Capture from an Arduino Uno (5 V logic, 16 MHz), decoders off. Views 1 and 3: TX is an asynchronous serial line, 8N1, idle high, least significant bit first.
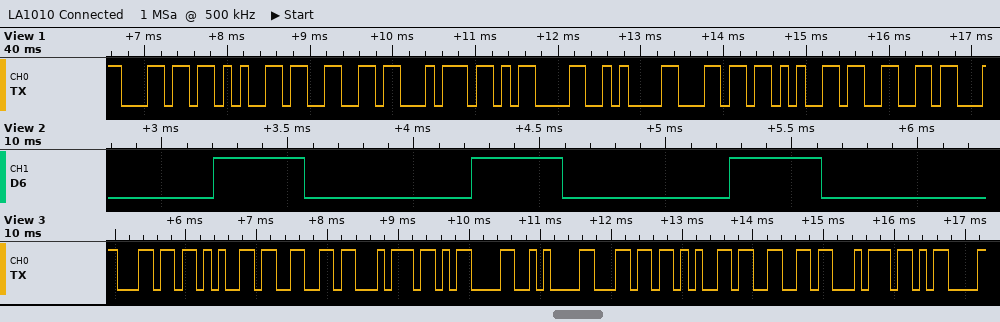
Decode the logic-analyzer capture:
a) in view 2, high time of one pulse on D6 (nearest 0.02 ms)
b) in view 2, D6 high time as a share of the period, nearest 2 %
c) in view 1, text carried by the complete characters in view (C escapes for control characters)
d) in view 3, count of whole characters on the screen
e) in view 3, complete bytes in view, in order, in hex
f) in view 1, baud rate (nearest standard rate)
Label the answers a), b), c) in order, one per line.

a) 0.36 ms
b) 36 %
c) "left\r\nlef"
d) 11
e) 6C 65 66 74 0D 0A 6C 65 66 74 0D
f) 9600 baud
